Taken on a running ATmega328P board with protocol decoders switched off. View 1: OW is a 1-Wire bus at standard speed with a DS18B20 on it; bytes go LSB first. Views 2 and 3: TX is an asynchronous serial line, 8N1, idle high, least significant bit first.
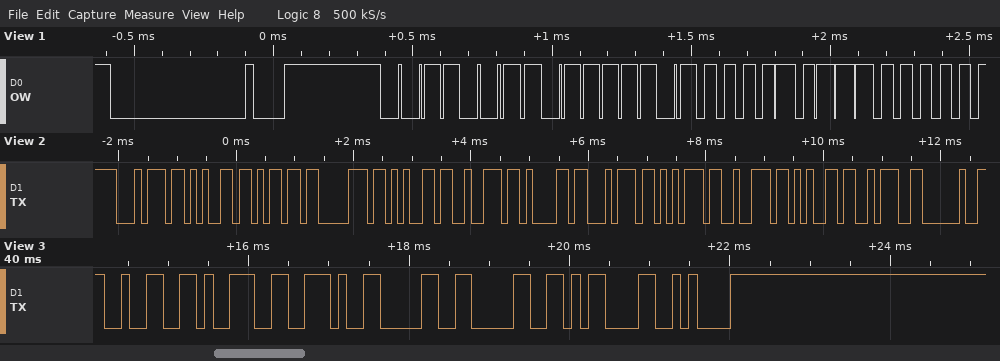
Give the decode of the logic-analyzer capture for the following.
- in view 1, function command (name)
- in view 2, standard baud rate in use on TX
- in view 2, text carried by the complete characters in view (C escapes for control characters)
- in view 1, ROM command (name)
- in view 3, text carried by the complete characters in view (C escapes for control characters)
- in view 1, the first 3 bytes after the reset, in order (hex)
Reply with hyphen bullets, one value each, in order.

- Read Scratchpad
- 9600 baud
- "temperature: "
- Skip ROM
- "29.00\r\n"
- CC BE D0
